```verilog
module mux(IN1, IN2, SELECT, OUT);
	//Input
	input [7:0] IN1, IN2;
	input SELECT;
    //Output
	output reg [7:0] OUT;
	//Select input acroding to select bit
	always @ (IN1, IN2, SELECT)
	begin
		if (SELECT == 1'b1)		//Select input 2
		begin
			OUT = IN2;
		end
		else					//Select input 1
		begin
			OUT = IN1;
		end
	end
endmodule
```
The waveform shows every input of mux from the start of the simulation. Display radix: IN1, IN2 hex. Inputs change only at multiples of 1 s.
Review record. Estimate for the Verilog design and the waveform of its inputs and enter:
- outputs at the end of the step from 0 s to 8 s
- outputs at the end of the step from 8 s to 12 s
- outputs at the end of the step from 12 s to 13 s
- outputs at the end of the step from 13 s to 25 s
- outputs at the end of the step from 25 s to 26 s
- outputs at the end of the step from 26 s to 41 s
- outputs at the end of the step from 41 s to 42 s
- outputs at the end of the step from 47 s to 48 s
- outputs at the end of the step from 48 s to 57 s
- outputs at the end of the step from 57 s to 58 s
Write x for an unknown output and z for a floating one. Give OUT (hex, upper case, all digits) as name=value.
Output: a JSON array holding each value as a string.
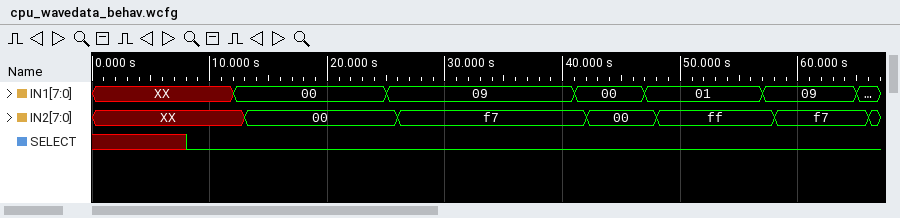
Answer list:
["OUT=x", "OUT=x", "OUT=00", "OUT=00", "OUT=09", "OUT=09", "OUT=00", "OUT=01", "OUT=01", "OUT=09"]
